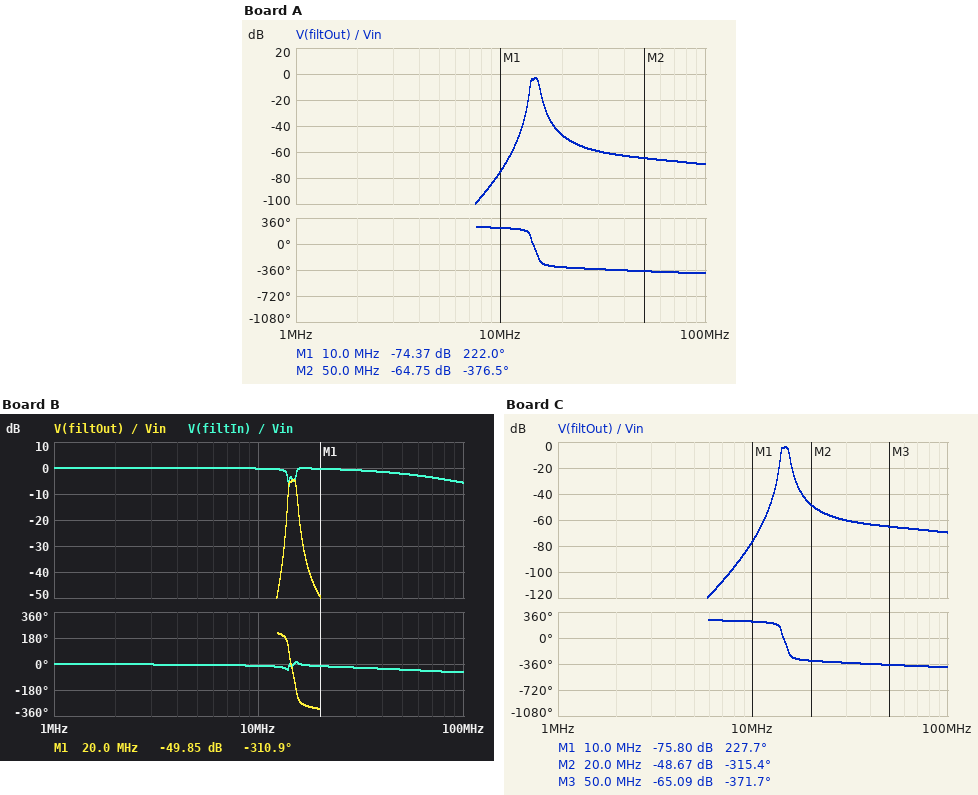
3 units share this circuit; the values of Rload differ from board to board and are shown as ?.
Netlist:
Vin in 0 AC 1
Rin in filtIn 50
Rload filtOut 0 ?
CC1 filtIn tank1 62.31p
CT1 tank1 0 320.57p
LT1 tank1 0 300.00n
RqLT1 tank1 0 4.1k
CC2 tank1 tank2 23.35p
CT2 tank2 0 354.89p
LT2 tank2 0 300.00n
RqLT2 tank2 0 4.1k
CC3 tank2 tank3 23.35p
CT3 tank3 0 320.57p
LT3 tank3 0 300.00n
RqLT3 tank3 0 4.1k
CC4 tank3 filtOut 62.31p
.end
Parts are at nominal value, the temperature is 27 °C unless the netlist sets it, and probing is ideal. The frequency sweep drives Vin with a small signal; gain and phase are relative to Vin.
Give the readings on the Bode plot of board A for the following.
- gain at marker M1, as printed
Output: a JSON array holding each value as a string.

["-74.37 dB"]
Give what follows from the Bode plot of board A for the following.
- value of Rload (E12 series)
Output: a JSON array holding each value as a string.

["150 Ω"]
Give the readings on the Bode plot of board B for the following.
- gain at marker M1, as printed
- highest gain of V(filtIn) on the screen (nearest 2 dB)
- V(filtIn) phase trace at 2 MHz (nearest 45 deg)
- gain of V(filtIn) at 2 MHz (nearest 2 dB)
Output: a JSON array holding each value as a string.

["-49.85 dB", "0 dB", "0 deg", "0 dB"]
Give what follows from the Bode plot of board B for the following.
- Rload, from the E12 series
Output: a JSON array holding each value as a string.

["100 Ω"]
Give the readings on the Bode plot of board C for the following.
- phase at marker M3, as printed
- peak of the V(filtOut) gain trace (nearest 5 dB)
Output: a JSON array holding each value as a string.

["-371.7 deg", "-5 dB"]
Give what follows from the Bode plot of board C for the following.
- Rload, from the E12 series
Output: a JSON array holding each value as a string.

["120 Ω"]
